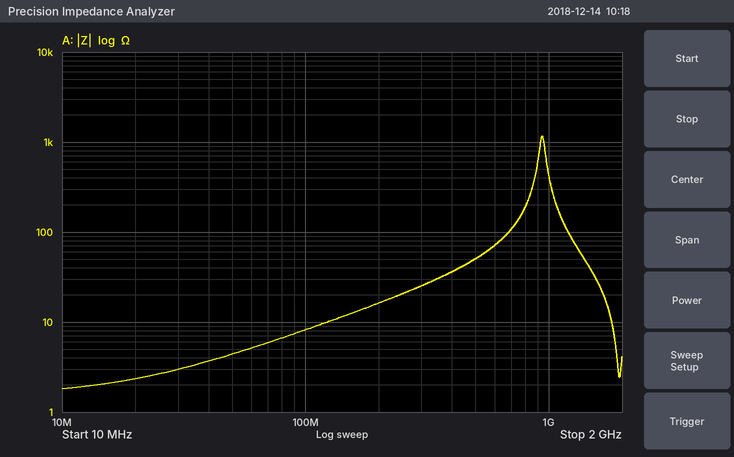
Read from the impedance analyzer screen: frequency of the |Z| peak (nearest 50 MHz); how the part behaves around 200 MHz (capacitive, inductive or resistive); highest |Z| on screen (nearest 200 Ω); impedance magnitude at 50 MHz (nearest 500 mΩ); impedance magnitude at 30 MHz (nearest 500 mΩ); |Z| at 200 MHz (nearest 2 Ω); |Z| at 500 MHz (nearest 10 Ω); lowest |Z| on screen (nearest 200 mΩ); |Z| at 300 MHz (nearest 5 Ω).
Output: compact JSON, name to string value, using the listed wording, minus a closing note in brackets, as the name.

{"frequency of the |Z| peak": "950 MHz", "how the part behaves around 200 MHz": "inductive", "highest |Z| on screen": "1.2 kΩ", "impedance magnitude at 50 MHz": "4.5 Ω", "impedance magnitude at 30 MHz": "3.0 Ω", "|Z| at 200 MHz": "16 Ω", "|Z| at 500 MHz": "50 Ω", "lowest |Z| on screen": "1.8 Ω", "|Z| at 300 MHz": "25 Ω"}
